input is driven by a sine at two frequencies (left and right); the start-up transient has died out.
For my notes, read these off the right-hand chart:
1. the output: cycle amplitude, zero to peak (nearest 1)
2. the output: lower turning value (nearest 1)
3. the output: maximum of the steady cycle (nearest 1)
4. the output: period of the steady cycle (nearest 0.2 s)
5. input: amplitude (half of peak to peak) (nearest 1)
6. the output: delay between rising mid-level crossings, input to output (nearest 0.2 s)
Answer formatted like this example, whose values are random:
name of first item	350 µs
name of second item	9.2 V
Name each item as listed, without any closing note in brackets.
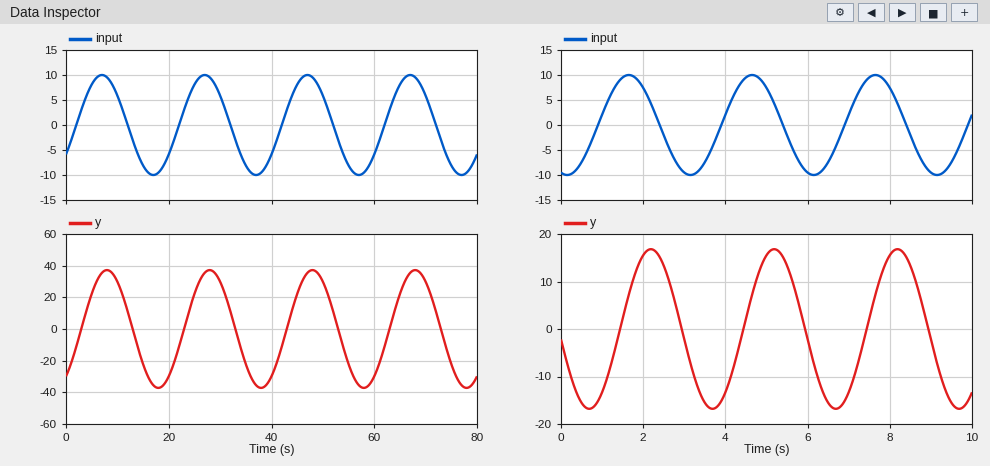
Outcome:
the output: cycle amplitude, zero to peak	17
the output: lower turning value	-17
the output: maximum of the steady cycle	17
the output: period of the steady cycle	3.0 s
input: amplitude (half of peak to peak)	10
the output: delay between rising mid-level crossings, input to output	0.6 s
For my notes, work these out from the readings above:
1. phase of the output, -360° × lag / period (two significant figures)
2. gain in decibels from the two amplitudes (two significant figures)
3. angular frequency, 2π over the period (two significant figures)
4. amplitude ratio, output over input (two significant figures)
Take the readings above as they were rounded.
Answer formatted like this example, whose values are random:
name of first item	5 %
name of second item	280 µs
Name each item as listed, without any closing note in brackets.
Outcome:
phase of the output, -360° × lag / period	-72°
gain in decibels from the two amplitudes	4.6 dB
angular frequency, 2π over the period	2.1 rad/s
amplitude ratio, output over input	1.7
